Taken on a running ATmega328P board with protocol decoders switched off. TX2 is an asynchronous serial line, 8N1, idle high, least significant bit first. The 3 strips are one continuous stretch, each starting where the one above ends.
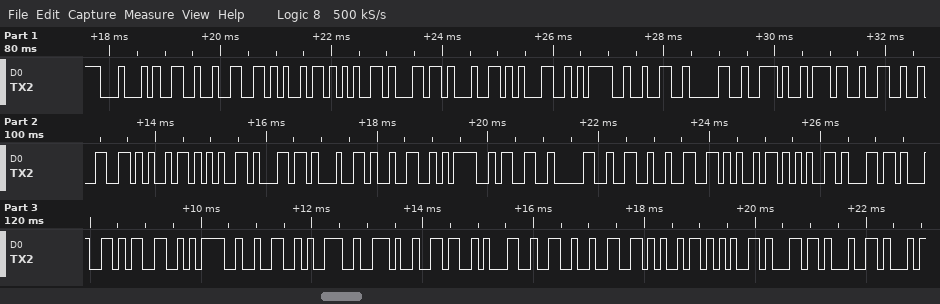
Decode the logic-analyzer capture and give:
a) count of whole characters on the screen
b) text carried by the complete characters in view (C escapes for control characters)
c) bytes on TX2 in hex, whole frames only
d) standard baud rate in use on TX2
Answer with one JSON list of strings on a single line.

["42", "\"D&field1=20.7&field2=30&field3=29.61&field\"", "0x44 0x26 0x66 0x69 0x65 0x6C 0x64 0x31 0x3D 0x32 0x30 0x2E 0x37 0x26 0x66 0x69 0x65 0x6C 0x64 0x32 0x3D 0x33 0x30 0x26 0x66 0x69 0x65 0x6C 0x64 0x33 0x3D 0x32 0x39 0x2E 0x36 0x31 0x26 0x66 0x69 0x65 0x6C 0x64", "9600 baud"]
